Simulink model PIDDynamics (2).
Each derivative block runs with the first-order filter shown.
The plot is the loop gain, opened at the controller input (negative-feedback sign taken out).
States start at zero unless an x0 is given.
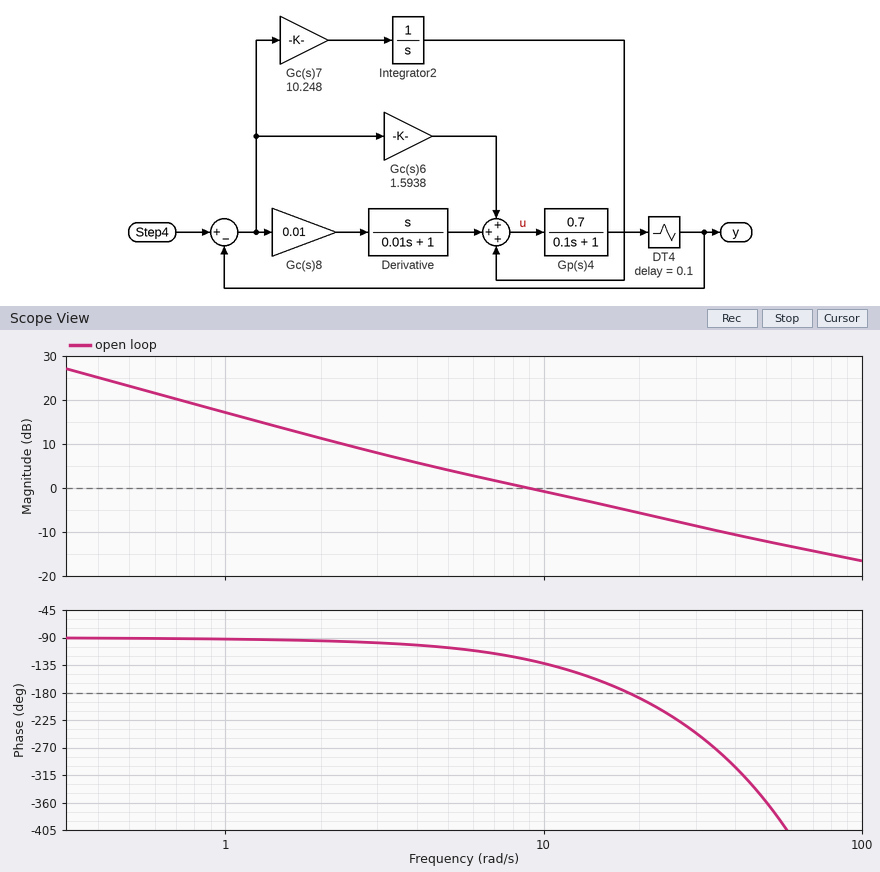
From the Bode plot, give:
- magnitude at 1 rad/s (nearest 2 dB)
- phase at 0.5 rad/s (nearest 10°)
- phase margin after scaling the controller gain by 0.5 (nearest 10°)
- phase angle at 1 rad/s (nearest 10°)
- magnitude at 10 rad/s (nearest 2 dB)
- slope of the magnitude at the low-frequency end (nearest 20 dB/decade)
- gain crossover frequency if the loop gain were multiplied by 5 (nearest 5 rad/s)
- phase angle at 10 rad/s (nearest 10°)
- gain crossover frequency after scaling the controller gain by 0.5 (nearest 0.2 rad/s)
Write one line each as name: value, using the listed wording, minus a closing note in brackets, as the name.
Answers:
magnitude at 1 rad/s: 18 dB
phase at 0.5 rad/s: -90°
phase margin after scaling the controller gain by 0.5: 80°
phase angle at 1 rad/s: -90°
magnitude at 10 rad/s: 0 dB
slope of the magnitude at the low-frequency end: -20 dB/decade
gain crossover frequency if the loop gain were multiplied by 5: 65 rad/s
phase angle at 10 rad/s: -130°
gain crossover frequency after scaling the controller gain by 0.5: 3.8 rad/s
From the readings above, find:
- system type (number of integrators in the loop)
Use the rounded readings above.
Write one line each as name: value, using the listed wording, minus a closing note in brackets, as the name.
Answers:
system type: 1
